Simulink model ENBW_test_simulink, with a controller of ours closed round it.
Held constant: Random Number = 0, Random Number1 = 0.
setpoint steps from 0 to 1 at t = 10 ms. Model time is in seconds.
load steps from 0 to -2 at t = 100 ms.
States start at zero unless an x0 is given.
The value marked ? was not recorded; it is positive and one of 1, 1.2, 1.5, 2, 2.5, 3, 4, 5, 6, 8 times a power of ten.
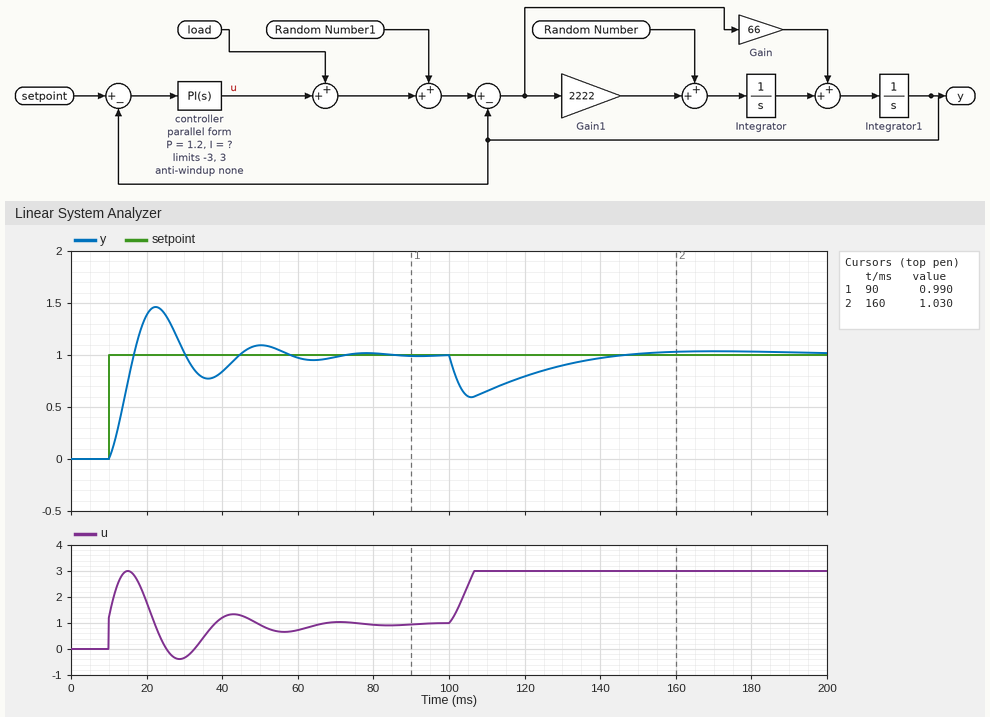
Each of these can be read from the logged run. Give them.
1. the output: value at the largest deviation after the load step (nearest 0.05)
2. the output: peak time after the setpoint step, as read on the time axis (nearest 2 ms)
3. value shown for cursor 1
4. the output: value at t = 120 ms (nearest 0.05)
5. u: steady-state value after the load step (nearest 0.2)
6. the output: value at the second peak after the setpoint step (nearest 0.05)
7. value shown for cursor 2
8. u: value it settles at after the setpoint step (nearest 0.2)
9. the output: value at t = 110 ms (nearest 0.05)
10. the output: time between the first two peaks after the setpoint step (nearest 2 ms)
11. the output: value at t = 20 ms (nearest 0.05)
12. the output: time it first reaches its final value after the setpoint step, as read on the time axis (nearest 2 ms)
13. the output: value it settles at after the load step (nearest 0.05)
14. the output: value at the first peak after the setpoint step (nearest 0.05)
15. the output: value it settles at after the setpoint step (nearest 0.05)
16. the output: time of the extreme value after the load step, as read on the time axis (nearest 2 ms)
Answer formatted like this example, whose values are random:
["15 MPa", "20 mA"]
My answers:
["0.60", "22 ms", "0.990", "0.80", "3.0", "1.10", "1.030", "1.0", "0.65", "28 ms", "1.40", "16 ms", "1.00", "1.45", "1.00", "106 ms"]
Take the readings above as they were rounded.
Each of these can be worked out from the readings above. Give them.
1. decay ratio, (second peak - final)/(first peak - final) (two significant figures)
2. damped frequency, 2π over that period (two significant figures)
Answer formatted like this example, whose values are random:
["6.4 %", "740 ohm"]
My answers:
["0.22", "0.22 rad/ms"]
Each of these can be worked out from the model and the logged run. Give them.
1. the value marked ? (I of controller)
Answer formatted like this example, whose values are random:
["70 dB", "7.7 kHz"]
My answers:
["800"]
